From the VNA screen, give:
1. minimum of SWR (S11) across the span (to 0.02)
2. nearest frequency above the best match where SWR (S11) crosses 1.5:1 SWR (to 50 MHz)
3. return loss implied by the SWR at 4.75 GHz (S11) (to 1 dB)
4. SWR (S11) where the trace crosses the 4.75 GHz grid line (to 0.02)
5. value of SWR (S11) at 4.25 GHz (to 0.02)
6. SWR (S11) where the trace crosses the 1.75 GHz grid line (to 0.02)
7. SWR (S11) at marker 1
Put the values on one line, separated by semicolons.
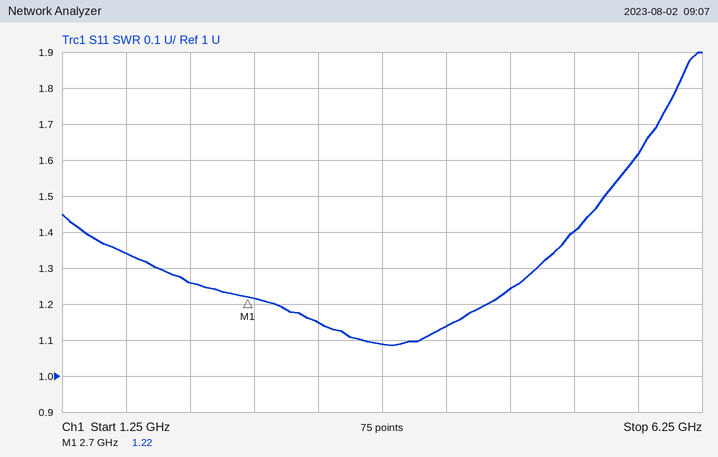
1.08; 5.50 GHz; 19 dB; 1.24; 1.14; 1.34; 1.22
